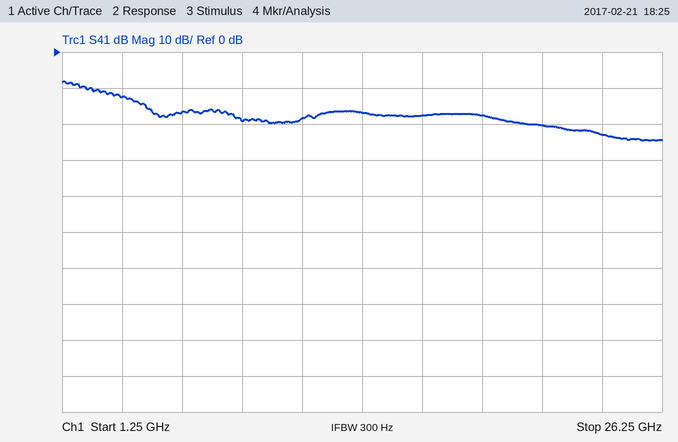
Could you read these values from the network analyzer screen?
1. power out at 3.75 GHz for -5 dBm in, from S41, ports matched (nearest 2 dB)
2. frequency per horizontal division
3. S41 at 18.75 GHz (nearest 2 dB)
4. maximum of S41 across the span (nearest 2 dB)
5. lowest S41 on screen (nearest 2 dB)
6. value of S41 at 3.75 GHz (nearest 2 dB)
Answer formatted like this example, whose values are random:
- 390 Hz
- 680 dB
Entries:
- -18 dBm
- 2.5 GHz
- -18 dB
- -8 dB
- -24 dB
- -12 dB
